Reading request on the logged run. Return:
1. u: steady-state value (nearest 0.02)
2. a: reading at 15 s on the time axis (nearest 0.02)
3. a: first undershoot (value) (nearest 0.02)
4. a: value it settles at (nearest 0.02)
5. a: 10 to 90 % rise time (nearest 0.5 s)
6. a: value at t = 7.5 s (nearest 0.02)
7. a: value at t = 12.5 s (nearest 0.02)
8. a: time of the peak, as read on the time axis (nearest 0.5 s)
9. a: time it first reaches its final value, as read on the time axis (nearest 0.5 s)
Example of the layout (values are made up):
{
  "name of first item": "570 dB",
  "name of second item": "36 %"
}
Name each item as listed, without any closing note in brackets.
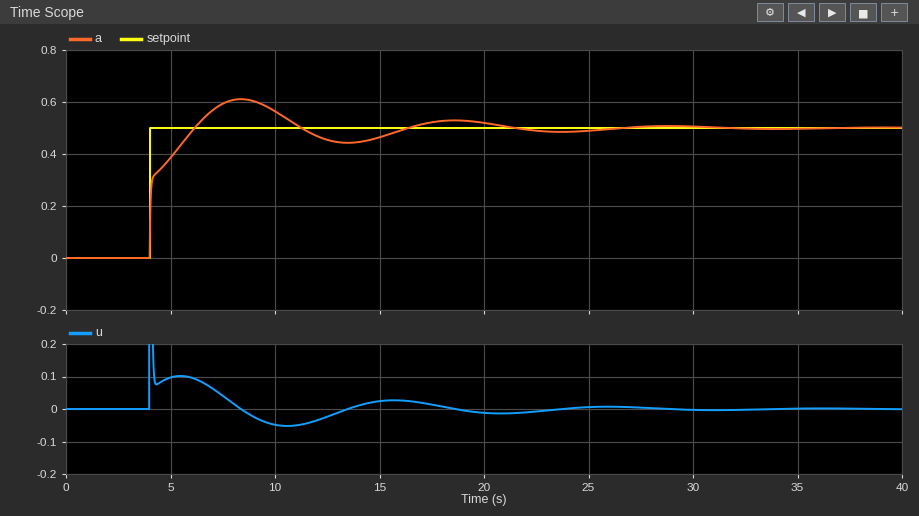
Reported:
{
  "u: steady-state value": "0.00",
  "a: reading at 15 s on the time axis": "0.46",
  "a: first undershoot (value)": "0.44",
  "a: value it settles at": "0.50",
  "a: 10 to 90 % rise time": "1.5 s",
  "a: value at t = 7.5 s": "0.60",
  "a: value at t = 12.5 s": "0.46",
  "a: time of the peak, as read on the time axis": "8.5 s",
  "a: time it first reaches its final value, as read on the time axis": "6.0 s"
}
